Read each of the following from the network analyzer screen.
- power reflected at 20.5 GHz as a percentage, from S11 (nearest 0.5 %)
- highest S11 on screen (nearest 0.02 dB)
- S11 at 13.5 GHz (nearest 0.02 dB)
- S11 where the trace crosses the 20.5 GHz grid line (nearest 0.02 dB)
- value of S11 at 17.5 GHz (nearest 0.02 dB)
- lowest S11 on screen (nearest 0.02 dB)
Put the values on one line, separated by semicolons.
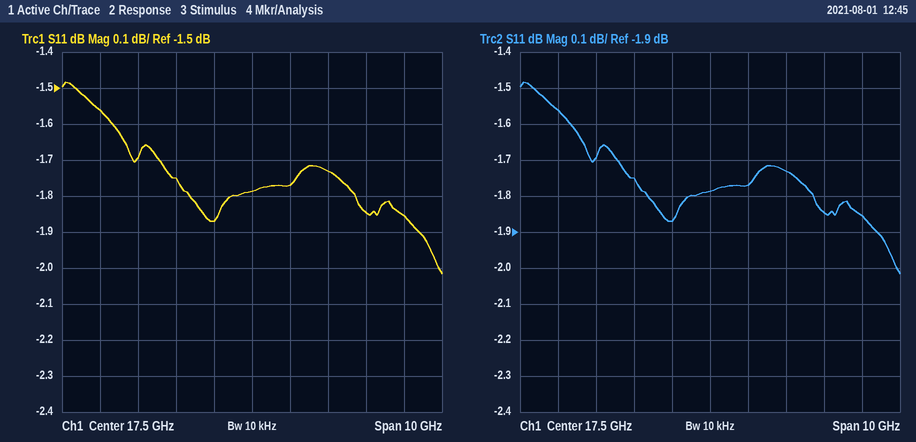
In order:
65.5 %; -1.48 dB; -1.56 dB; -1.84 dB; -1.78 dB; -2.02 dB
